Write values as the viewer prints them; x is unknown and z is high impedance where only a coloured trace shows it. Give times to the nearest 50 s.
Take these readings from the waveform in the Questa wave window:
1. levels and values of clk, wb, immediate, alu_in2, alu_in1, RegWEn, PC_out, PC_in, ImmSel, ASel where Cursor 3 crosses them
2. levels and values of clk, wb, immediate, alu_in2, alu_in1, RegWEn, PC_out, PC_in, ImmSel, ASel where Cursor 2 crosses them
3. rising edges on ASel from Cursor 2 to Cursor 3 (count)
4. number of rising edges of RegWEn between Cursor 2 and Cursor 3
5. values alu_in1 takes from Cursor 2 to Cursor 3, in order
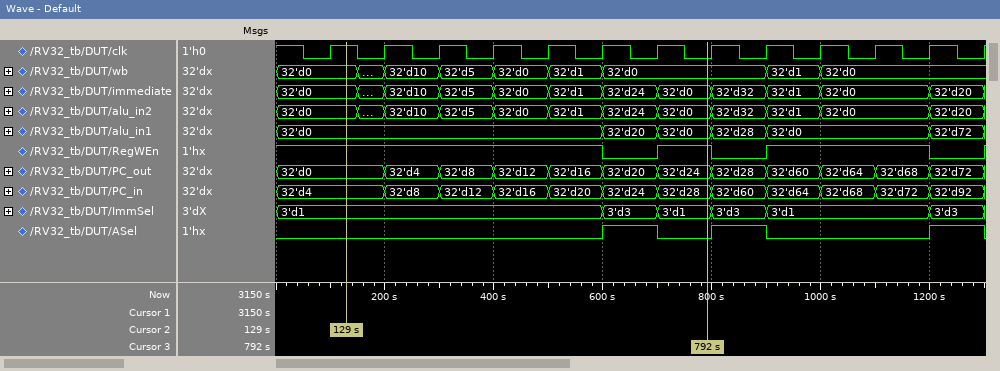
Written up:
clk=0, wb=32'd0, immediate=32'd0, alu_in2=32'd0, alu_in1=32'd0, RegWEn=1, PC_out=32'd24, PC_in=32'd28, ImmSel=3'd1, ASel=0
clk=1, wb=32'd0, immediate=32'd0, alu_in2=32'd0, alu_in1=32'd0, RegWEn=1, PC_out=32'd0, PC_in=32'd4, ImmSel=3'd1, ASel=0
1
1
32'd0, 32'd20, 32'd0
